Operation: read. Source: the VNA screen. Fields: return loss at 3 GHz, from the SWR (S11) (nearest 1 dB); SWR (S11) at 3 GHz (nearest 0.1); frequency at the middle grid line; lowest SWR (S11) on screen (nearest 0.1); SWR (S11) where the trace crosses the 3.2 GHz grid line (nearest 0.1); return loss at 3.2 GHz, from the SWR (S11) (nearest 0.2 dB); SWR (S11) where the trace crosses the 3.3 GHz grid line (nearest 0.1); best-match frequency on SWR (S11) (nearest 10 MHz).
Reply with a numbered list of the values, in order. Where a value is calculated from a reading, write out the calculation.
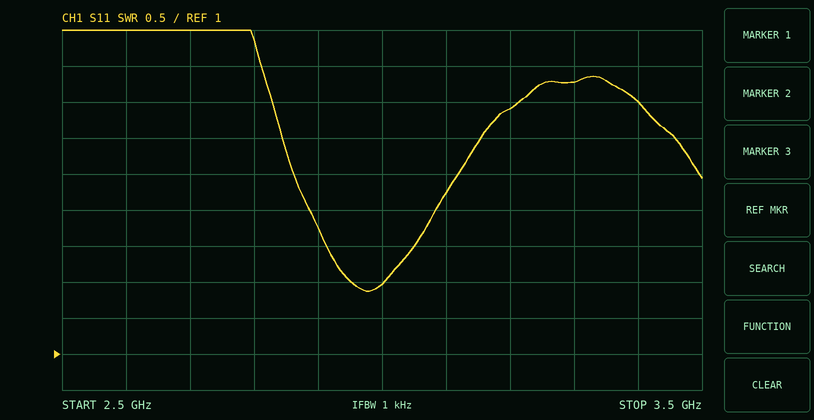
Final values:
1. −20 log10((2 − 1)/(2 + 1)) ≈ 10 dB
2. 2.0
3. 3 GHz
4. 1.9
5. 4.4
6. −20 log10((4.4 − 1)/(4.4 + 1)) ≈ 4.0 dB
7. 4.8
8. 2.98 GHz
